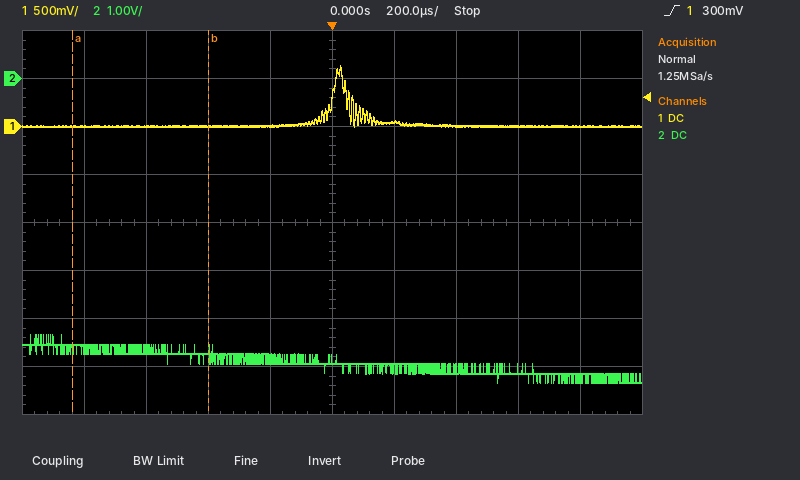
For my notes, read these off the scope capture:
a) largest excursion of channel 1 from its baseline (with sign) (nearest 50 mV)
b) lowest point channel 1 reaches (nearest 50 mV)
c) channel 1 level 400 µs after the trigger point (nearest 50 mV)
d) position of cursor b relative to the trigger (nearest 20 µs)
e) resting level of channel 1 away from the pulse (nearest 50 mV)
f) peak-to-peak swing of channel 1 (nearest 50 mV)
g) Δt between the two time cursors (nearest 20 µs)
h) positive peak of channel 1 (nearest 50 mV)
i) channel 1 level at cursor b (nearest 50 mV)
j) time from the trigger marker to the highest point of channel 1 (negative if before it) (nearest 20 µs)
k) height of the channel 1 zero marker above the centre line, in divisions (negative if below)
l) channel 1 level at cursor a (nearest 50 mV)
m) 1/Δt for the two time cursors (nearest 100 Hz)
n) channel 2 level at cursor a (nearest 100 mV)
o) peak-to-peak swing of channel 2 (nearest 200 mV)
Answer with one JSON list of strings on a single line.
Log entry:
["+650 mV", "0 mV", "0 mV", "-400 µs", "0 mV", "650 mV", "440 µs", "650 mV", "0 mV", "+20 µs", "+2.0 div", "0 mV", "2.3 kHz", "-5.6 V", "1.0 V"]
